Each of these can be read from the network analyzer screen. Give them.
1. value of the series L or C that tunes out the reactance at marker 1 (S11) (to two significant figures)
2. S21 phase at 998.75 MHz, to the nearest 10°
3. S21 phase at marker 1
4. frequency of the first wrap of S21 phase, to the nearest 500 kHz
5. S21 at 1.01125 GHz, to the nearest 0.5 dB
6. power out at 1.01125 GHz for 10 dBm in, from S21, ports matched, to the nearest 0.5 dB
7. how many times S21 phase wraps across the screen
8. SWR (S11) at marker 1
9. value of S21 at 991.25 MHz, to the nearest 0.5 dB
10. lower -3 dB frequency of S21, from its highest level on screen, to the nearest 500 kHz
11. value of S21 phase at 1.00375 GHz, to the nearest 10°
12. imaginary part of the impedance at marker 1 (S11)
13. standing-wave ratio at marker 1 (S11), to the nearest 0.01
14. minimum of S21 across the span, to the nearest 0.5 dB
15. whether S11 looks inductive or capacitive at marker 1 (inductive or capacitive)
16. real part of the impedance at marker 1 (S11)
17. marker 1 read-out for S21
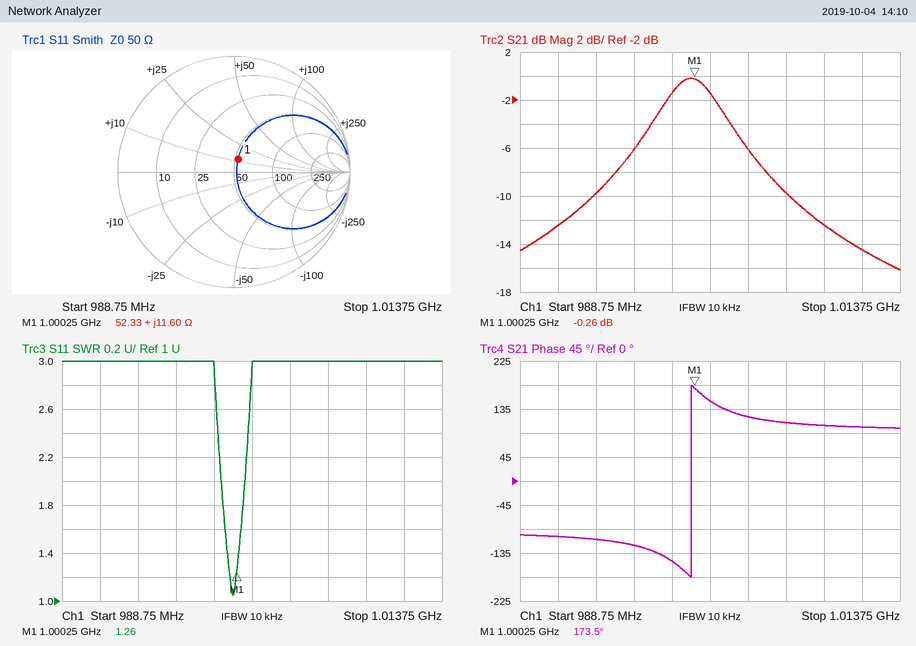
14 pF
-150°
173.5°
1.0000 GHz
-14.5 dB
-4.5 dBm
1
1.26
-12.5 dB
998.0 MHz
120°
+11.60 Ω
1.26
-16.0 dB
inductive
52.33 Ω
-0.26 dB
